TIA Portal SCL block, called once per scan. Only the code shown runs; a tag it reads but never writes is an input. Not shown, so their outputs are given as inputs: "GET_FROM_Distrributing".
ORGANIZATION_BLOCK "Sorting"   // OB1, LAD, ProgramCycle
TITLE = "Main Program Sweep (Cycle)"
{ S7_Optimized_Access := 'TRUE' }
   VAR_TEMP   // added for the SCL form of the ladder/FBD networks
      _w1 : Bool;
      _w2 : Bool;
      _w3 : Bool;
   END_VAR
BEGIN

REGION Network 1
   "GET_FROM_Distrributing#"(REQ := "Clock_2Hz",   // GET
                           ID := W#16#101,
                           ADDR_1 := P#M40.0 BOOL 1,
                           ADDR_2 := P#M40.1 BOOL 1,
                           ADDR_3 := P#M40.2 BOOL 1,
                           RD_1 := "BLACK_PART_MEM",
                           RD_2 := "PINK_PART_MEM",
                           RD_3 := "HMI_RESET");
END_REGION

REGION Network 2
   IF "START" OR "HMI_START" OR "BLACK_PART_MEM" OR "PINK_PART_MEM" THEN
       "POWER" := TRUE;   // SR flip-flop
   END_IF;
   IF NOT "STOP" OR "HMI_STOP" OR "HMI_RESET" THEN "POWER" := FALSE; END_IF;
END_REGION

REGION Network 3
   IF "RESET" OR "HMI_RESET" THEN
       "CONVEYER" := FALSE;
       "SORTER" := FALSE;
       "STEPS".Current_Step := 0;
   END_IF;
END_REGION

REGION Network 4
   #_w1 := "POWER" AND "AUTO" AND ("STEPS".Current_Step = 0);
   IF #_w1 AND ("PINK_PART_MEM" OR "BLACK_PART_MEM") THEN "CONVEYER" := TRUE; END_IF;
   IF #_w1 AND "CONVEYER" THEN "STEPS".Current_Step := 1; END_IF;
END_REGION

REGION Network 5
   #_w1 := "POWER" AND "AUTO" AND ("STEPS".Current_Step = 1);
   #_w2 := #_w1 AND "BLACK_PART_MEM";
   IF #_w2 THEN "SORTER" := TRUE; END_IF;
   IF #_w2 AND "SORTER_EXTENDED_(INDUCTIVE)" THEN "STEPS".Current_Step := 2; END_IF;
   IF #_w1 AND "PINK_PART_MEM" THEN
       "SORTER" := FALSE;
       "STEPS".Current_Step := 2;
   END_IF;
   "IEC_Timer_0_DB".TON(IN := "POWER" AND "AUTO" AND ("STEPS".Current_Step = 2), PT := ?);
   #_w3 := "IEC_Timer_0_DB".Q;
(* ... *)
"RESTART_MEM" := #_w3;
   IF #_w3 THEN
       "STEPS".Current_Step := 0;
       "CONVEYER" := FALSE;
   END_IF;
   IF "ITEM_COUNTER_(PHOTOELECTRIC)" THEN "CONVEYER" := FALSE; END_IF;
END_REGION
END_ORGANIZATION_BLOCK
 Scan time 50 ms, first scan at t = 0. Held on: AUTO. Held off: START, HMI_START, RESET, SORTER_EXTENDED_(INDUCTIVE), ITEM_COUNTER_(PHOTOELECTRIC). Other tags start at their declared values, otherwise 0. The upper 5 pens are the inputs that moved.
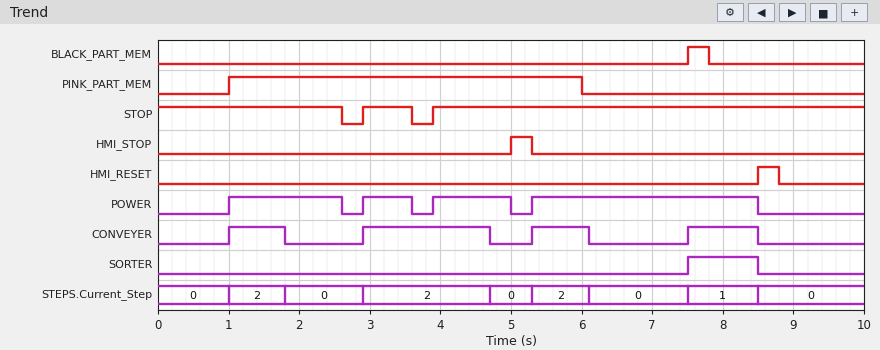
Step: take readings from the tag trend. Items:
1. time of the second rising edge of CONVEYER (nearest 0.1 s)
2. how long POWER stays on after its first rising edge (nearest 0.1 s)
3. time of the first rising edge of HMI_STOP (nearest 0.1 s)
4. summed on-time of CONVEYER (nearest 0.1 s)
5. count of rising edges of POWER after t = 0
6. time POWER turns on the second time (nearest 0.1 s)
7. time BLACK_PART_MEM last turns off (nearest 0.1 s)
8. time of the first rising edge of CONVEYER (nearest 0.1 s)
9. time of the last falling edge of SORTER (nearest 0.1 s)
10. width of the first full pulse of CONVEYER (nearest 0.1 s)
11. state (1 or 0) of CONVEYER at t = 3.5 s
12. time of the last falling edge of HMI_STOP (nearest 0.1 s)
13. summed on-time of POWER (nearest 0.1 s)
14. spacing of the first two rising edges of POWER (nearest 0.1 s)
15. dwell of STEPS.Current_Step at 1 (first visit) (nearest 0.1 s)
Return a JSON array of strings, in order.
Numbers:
["2.9 s", "1.6 s", "5.0 s", "4.4 s", "4", "2.9 s", "7.8 s", "1.0 s", "8.5 s", "0.8 s", "1", "5.3 s", "6.6 s", "1.9 s", "1.0 s"]
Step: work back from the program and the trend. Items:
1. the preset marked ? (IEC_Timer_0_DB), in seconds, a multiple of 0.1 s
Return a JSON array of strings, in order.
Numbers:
["0.8 s"]
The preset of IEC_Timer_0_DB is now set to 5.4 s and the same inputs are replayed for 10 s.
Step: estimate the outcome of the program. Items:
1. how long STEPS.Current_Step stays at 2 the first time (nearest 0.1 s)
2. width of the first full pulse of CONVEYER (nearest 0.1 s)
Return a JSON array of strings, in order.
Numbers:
["7.5 s", "7.5 s"]
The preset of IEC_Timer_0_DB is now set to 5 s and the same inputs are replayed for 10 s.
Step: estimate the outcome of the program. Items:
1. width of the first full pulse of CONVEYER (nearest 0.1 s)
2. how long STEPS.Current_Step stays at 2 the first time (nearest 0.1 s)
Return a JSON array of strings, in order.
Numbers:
["7.5 s", "7.5 s"]
